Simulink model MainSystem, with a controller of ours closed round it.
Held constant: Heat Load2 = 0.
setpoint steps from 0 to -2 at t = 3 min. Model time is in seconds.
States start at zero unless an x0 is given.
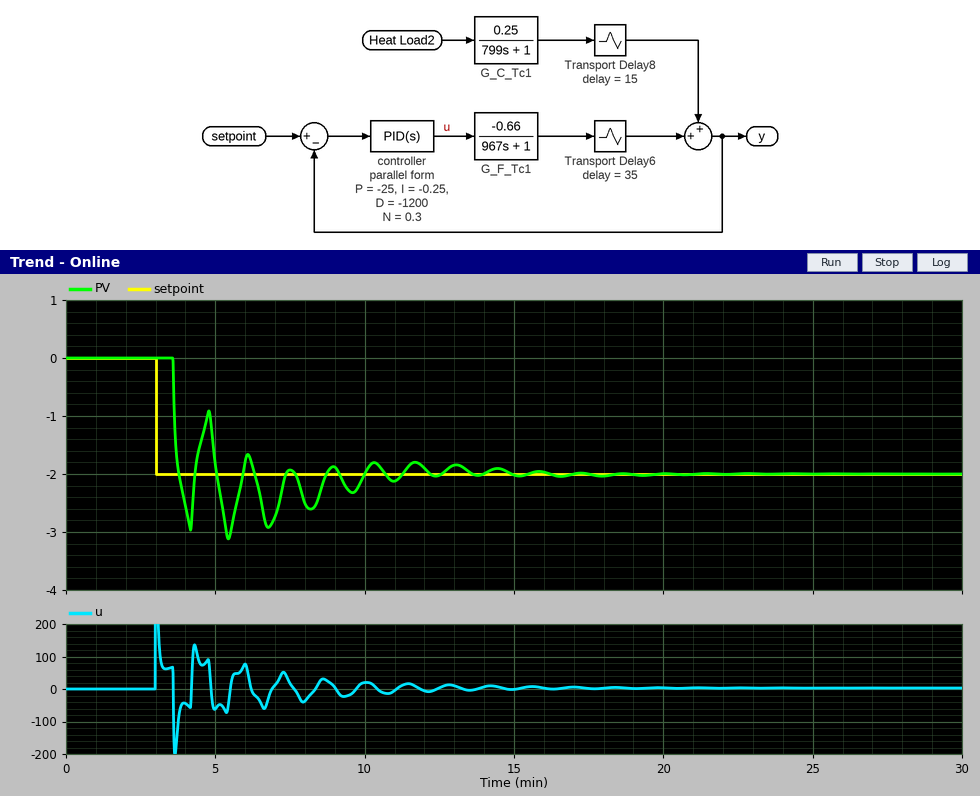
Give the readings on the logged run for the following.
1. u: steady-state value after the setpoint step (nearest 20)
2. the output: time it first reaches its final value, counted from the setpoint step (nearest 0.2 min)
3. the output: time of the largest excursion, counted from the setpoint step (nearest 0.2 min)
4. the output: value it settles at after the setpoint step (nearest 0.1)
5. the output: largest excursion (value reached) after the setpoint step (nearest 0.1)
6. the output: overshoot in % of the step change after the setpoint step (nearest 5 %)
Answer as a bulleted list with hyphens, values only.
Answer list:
- 0
- 0.8 min
- 2.4 min
- -2.0
- -3.1
- 55 %
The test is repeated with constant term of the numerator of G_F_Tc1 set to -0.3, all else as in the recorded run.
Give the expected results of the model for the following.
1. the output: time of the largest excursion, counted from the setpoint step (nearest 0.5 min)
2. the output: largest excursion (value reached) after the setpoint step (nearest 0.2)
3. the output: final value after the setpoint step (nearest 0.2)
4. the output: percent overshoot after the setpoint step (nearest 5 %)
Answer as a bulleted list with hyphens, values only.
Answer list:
- 5.5 min
- -2.6
- -2.0
- 30 %
